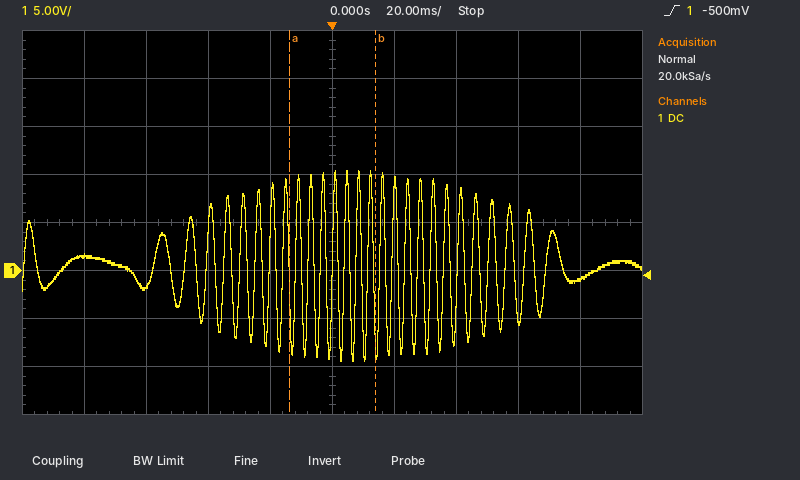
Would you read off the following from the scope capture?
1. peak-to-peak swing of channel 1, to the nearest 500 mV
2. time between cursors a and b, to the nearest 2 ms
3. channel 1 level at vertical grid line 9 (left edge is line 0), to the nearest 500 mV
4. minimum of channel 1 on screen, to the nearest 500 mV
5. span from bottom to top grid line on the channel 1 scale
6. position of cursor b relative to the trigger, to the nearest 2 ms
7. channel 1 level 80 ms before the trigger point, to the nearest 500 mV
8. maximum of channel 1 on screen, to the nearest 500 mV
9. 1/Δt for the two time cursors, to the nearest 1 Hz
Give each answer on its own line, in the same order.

20.0 V
28 ms
-1.0 V
-9.5 V
40 V
+14 ms
1.5 V
10.5 V
36 Hz
